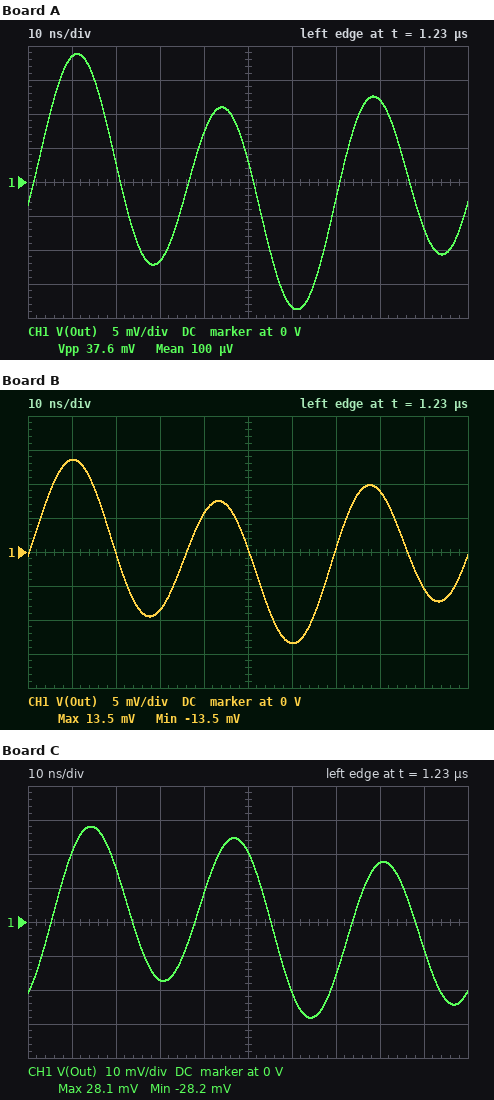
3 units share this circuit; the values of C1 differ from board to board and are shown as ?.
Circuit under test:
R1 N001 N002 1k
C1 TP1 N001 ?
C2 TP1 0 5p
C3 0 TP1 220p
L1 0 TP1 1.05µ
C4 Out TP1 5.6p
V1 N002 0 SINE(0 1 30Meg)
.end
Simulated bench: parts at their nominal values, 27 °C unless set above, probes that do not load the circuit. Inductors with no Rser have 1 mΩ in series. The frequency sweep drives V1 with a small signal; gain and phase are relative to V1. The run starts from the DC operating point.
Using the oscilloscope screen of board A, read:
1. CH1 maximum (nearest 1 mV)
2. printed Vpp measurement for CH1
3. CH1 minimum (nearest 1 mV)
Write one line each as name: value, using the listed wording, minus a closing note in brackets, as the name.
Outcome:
CH1 maximum: 19 mV
printed Vpp measurement for CH1: 37.6 mV
CH1 minimum: -19 mV
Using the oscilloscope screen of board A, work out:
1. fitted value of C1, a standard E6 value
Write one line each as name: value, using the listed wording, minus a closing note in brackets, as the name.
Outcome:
fitted value of C1, a standard E6 value: 3.3 pF
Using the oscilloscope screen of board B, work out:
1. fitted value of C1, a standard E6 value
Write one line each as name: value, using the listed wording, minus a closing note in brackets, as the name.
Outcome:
fitted value of C1, a standard E6 value: 2.2 pF
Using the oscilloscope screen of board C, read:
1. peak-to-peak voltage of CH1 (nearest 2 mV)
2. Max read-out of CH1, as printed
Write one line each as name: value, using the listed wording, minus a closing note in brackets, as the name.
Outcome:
peak-to-peak voltage of CH1: 56 mV
Max read-out of CH1, as printed: 28.1 mV
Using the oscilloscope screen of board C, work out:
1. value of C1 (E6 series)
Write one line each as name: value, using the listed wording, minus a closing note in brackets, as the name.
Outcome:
value of C1: 10 pF
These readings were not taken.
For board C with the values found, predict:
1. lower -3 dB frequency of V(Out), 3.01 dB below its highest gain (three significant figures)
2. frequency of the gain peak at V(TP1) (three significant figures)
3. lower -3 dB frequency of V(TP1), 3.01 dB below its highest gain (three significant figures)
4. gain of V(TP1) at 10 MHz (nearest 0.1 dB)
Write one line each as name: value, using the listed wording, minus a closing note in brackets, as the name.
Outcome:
lower -3 dB frequency of V(Out), 3.01 dB below its highest gain: 10.1 MHz
frequency of the gain peak at V(TP1): 10.2 MHz
lower -3 dB frequency of V(TP1), 3.01 dB below its highest gain: 10.1 MHz
gain of V(TP1) at 10 MHz: -1.6 dB
